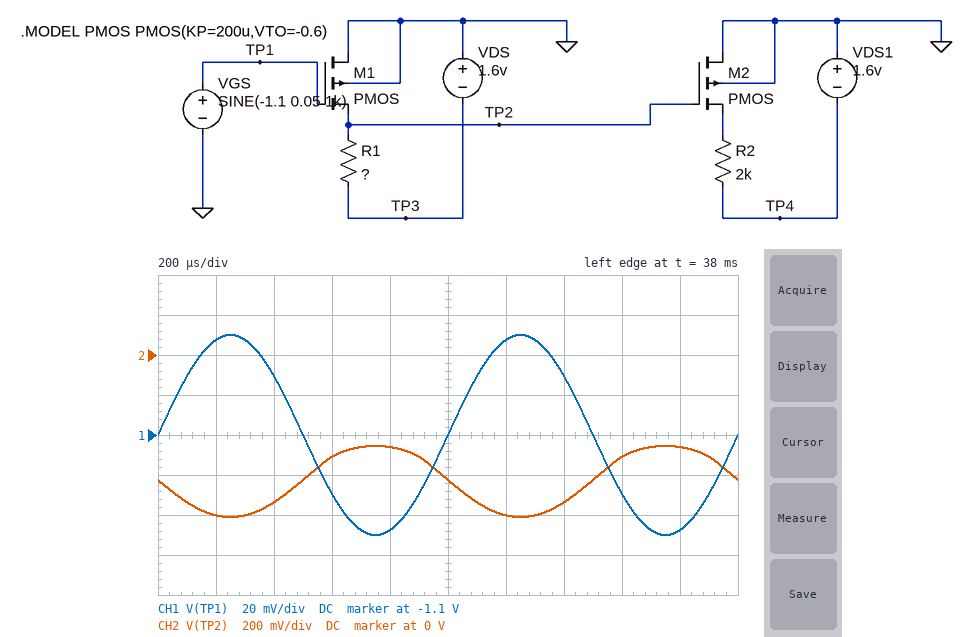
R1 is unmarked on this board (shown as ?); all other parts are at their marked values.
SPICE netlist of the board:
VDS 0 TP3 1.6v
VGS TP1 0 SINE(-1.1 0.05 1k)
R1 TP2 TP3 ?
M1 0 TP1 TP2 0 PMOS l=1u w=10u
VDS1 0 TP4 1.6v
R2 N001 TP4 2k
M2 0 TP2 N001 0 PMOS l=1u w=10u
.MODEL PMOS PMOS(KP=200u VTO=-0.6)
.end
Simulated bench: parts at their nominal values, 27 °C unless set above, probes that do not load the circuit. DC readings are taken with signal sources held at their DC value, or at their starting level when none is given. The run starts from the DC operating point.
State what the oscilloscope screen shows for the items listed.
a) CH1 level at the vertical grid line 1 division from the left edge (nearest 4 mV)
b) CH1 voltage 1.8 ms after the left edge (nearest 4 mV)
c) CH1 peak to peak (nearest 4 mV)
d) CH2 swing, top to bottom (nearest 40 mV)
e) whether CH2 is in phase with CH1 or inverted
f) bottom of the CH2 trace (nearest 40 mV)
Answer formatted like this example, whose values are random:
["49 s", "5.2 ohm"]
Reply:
["-1.052 V", "-1.148 V", "100 mV", "360 mV", "inverted", "-800 mV"]
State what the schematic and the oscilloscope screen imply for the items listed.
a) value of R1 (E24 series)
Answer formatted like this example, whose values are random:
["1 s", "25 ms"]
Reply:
["3.9 kΩ"]
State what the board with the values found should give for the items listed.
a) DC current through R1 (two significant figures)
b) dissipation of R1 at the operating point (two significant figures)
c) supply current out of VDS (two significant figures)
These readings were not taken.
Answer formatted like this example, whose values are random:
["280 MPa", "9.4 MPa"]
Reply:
["250 µA", "240 µW", "250 µA"]
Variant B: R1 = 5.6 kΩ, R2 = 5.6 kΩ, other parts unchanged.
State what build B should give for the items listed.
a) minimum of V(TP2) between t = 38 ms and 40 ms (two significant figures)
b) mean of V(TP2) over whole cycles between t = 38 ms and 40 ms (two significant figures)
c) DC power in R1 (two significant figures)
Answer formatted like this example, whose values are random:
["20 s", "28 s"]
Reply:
["-470 mV", "-360 mV", "280 µW"]
